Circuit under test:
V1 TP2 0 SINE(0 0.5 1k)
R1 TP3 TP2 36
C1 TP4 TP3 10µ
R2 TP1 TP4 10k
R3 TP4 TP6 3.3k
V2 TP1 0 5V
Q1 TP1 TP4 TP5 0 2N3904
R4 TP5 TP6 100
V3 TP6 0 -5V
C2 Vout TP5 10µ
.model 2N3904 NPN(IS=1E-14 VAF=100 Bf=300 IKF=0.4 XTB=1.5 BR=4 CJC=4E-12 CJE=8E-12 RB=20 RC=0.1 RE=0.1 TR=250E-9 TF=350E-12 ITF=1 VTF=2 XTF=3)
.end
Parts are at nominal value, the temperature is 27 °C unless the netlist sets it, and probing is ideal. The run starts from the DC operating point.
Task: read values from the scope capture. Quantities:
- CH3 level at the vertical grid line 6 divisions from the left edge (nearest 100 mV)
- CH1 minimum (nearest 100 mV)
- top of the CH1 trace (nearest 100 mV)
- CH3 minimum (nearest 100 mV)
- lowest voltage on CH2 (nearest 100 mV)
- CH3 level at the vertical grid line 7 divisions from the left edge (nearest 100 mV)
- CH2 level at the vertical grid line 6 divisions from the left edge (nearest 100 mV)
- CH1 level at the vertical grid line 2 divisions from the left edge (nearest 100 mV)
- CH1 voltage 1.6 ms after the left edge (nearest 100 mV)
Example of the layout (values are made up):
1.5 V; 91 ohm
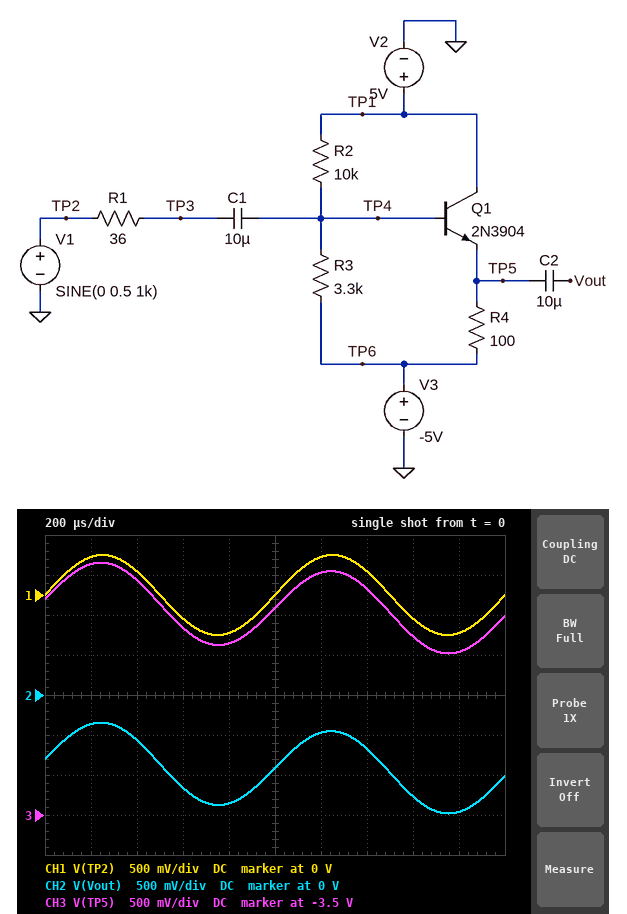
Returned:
-500 mV; -500 mV; 500 mV; -1.5 V; -1.5 V; -700 mV; -500 mV; 300 mV; -300 mV
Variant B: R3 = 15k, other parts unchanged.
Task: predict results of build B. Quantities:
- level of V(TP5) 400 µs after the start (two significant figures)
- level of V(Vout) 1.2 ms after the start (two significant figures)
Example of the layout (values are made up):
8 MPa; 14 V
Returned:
-470 mV; -290 mV
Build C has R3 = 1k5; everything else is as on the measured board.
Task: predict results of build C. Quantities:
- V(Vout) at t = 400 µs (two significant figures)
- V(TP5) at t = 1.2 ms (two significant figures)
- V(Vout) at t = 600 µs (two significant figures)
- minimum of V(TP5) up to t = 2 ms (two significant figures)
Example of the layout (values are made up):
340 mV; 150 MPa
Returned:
-700 mV; -730 mV; -1.3 V; -1.8 V
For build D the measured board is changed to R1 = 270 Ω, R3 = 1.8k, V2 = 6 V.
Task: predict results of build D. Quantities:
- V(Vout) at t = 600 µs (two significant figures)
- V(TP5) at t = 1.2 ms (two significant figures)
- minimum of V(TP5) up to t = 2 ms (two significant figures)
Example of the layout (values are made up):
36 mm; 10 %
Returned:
-1.6 V; -1.1 V; -2.0 V
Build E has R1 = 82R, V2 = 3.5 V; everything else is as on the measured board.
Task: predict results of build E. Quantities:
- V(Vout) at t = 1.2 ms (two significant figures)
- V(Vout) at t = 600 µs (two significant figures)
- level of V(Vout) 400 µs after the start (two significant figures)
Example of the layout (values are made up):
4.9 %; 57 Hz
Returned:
-550 mV; -1.2 V; -640 mV
